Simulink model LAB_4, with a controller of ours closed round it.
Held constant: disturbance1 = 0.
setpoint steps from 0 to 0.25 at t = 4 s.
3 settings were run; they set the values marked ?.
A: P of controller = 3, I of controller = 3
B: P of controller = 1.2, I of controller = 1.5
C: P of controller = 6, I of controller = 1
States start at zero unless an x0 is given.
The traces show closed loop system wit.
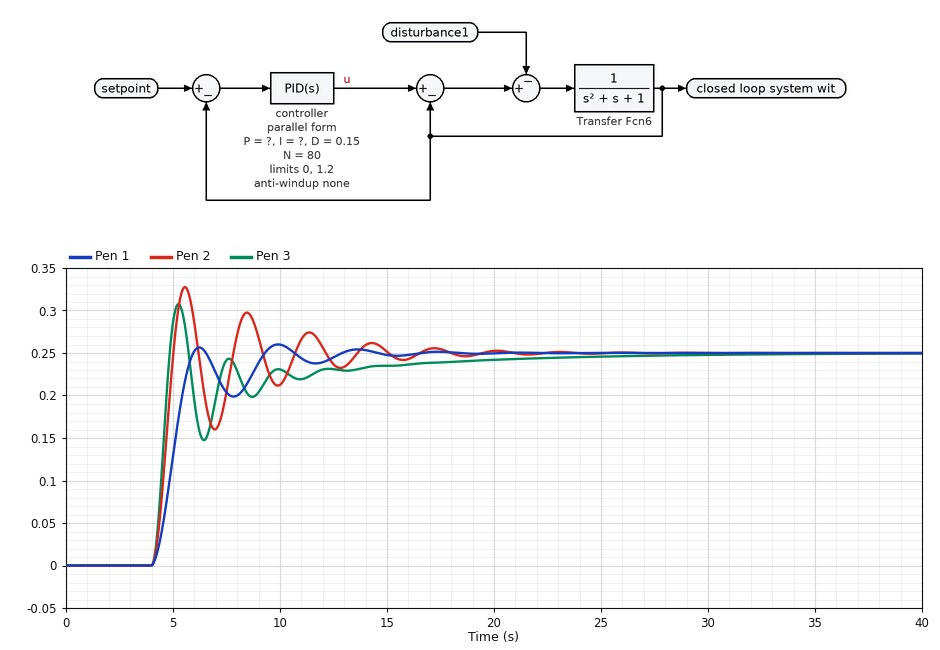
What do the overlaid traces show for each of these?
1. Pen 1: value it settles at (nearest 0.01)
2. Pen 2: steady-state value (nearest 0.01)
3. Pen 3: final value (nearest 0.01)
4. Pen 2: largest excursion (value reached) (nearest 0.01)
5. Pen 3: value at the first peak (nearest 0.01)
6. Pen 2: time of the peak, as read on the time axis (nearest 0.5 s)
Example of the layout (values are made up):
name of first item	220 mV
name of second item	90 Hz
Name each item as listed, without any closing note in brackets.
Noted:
Pen 1: value it settles at	0.25
Pen 2: steady-state value	0.25
Pen 3: final value	0.25
Pen 2: largest excursion (value reached)	0.33
Pen 3: value at the first peak	0.31
Pen 2: time of the peak, as read on the time axis	5.5 s
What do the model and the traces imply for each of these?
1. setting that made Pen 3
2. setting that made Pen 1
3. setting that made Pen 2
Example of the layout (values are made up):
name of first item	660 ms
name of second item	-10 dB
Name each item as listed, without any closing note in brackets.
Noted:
setting that made Pen 3	C
setting that made Pen 1	B
setting that made Pen 2	A
